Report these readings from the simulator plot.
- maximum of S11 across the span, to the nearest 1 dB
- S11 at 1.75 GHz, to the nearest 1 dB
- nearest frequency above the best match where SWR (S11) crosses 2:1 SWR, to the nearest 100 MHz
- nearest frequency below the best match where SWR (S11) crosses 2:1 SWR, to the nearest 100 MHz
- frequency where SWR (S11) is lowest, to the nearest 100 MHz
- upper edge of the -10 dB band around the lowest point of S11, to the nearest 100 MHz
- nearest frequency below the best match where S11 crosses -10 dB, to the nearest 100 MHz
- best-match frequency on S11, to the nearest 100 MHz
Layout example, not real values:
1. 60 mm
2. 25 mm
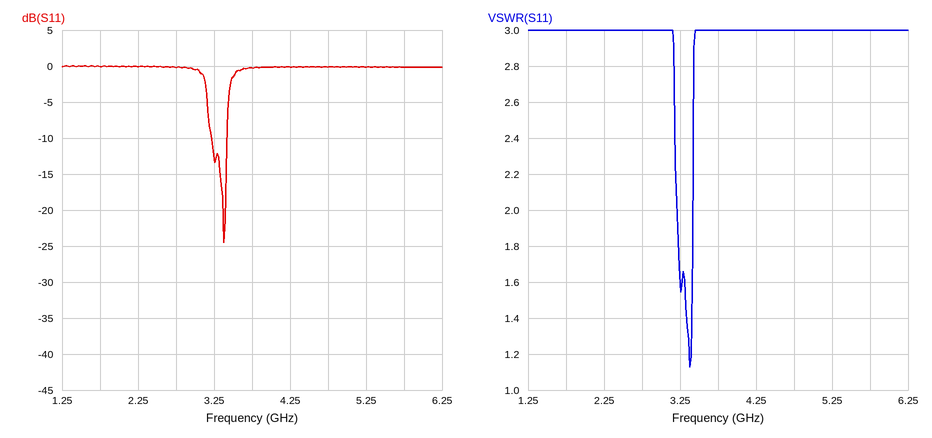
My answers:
1. 0 dB
2. 0 dB
3. 3.4 GHz
4. 3.2 GHz
5. 3.4 GHz
6. 3.4 GHz
7. 3.2 GHz
8. 3.4 GHz
